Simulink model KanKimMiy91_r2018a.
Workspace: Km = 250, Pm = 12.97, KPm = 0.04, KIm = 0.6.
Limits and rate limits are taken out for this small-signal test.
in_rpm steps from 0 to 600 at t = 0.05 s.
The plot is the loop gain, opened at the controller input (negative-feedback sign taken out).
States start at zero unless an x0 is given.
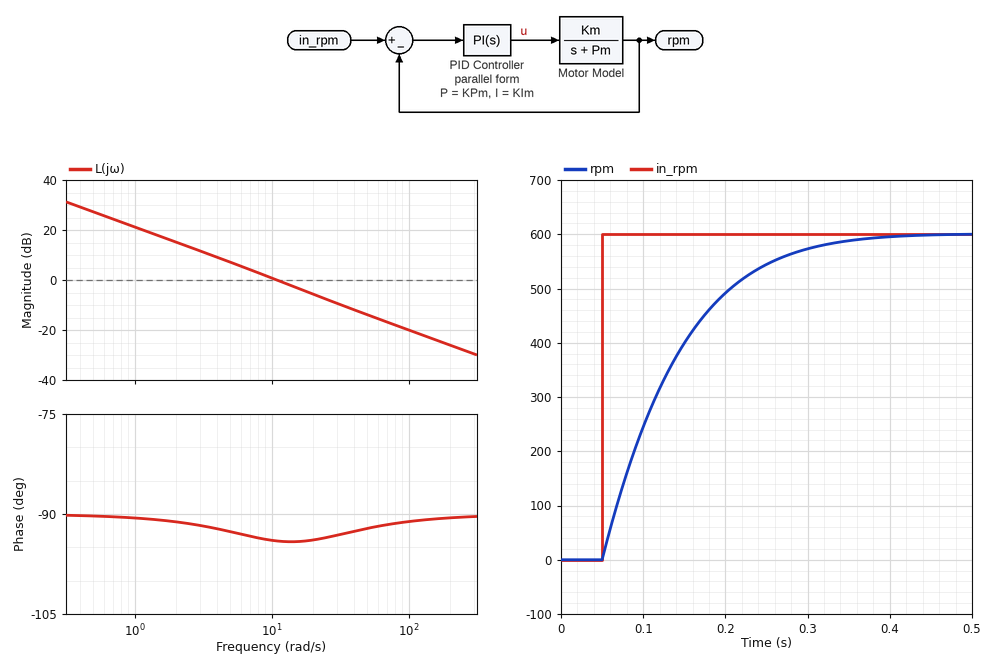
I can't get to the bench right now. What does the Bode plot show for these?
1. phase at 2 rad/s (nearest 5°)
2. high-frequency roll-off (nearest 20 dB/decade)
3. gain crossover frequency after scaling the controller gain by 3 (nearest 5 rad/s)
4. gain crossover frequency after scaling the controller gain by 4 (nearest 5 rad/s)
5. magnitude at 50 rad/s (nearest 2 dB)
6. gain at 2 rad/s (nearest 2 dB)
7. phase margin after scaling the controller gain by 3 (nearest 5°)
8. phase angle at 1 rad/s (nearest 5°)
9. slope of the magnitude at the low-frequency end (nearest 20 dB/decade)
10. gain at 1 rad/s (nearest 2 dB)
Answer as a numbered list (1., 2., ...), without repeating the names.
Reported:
1. -90°
2. -20 dB/decade
3. 30 rad/s
4. 40 rad/s
5. -14 dB
6. 16 dB
7. 85°
8. -90°
9. -20 dB/decade
10. 22 dB
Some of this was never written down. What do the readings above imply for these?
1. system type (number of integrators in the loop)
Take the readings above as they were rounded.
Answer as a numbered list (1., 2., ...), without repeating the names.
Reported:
1. 1
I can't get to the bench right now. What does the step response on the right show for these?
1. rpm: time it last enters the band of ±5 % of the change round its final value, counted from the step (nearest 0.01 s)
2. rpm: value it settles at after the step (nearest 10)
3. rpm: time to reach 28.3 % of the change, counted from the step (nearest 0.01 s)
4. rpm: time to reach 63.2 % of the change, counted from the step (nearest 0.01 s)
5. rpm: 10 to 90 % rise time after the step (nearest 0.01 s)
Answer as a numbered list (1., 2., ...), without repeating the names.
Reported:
1. 0.24 s
2. 600
3. 0.03 s
4. 0.09 s
5. 0.18 s
